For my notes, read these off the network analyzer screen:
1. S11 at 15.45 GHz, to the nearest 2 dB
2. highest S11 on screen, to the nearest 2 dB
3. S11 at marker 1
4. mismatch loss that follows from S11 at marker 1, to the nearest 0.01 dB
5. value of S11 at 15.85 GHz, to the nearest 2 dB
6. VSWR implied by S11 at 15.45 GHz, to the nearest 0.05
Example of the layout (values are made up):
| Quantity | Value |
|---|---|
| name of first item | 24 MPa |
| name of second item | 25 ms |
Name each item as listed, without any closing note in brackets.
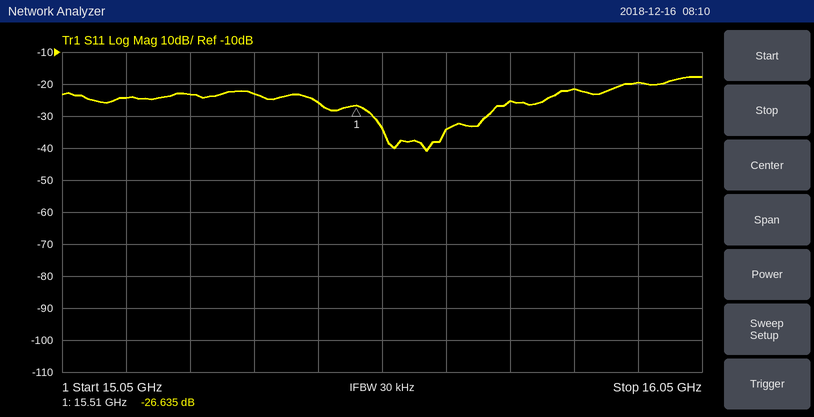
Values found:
| Quantity | Value |
|---|---|
| S11 at 15.45 GHz, to the nearest 2 dB | -26 dB |
| highest S11 on screen, to the nearest 2 dB | -18 dB |
| S11 at marker 1 | -26.635 dB |
| mismatch loss that follows from S11 at marker 1, to the nearest 0.01 dB | 0.01 dB |
| value of S11 at 15.85 GHz, to the nearest 2 dB | -22 dB |
| VSWR implied by S11 at 15.45 GHz, to the nearest 0.05 | 1.10 |
